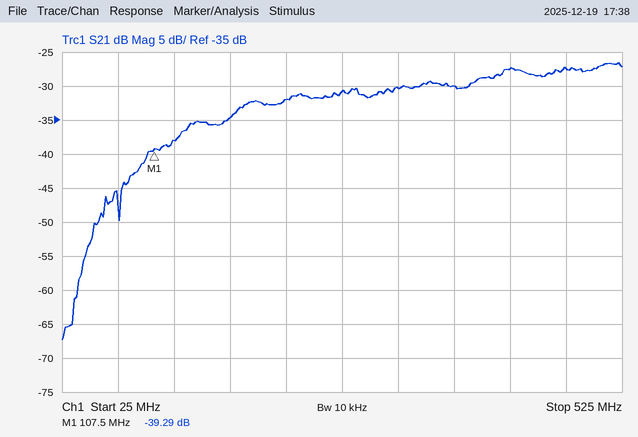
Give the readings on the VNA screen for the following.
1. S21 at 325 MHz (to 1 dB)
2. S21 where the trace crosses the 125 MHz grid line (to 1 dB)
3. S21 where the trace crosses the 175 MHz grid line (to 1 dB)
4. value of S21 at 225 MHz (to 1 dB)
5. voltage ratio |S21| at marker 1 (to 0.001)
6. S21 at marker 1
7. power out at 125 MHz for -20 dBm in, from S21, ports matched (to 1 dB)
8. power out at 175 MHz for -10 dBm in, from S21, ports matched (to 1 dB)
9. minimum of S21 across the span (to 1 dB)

-30 dB
-38 dB
-35 dB
-32 dB
0.011
-39.29 dB
-58 dBm
-45 dBm
-67 dB
